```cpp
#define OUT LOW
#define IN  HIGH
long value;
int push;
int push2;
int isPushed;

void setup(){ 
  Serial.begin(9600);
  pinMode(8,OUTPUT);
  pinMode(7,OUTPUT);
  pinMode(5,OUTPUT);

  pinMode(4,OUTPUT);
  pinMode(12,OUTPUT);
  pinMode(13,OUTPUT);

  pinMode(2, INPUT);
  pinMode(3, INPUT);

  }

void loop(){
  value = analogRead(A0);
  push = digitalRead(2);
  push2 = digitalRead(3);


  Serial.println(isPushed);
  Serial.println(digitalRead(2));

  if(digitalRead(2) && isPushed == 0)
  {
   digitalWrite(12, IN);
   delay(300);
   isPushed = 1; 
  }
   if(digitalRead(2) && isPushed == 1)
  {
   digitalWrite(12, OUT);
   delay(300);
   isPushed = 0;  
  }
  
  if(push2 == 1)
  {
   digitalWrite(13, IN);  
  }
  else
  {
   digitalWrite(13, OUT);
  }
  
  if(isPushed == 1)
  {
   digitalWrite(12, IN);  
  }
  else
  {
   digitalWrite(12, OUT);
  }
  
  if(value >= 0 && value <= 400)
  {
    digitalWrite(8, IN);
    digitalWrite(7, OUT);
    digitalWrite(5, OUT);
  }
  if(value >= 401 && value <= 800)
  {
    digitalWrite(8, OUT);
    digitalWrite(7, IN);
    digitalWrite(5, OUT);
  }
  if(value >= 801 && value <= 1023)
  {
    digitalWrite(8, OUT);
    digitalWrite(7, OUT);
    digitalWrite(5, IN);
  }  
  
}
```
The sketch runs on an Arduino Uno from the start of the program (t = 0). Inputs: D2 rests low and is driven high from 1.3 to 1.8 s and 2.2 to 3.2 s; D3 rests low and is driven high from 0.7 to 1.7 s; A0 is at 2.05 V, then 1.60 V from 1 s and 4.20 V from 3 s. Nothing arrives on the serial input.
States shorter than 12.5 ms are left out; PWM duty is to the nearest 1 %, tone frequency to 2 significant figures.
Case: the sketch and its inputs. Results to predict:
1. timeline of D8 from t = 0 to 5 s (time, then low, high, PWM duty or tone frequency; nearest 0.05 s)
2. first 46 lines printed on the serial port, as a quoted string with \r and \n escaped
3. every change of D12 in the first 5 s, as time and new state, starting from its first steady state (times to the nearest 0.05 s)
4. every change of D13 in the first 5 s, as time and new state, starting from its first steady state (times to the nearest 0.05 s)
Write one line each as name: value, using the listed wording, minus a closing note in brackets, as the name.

timeline of D8 from t = 0 to 5 s: 0 s low; 1 s high; 3.4 s low
first 46 lines printed on the serial port, as a quoted string with \r and \n escaped: "0\r\n0\r\n0\r\n0\r\n0\r\n0\r\n0\r\n0\r\n0\r\n0\r\n0\r\n0\r\n0\r\n0\r\n0\r\n0\r\n0\r\n0\r\n0\r\n0\r\n0\r\n0\r\n0\r\n0\r\n0\r\n0\r\n0\r\n0\r\n0\r\n0\r\n0\r\n0\r\n0\r\n0\r\n0\r\n0\r\n0\r\n0\r\n0\r\n0\r\n0\r\n0\r\n0\r\n0\r\n0\r\n0\r\n"
every change of D12 in the first 5 s, as time and new state, starting from its first steady state: 0 s low; 1.3 s high; 1.6 s low; 2.2 s high; 2.5 s low; 2.8 s high; 3.1 s low
every change of D13 in the first 5 s, as time and new state, starting from its first steady state: 0 s low; 0.7 s high; 1.9 s low
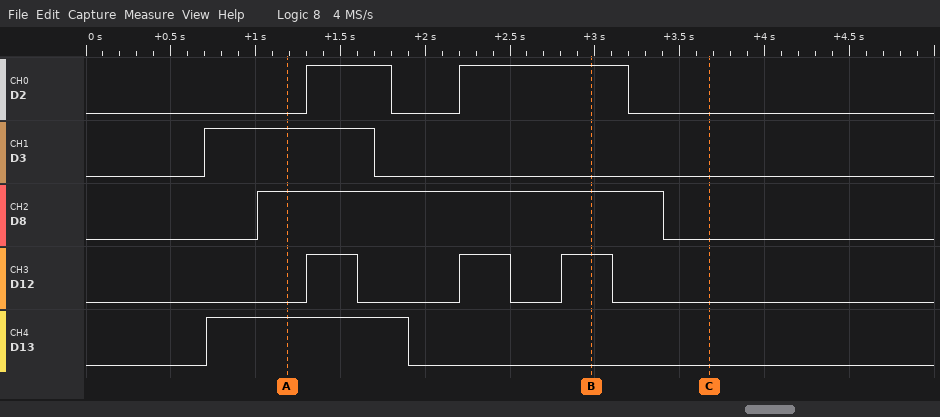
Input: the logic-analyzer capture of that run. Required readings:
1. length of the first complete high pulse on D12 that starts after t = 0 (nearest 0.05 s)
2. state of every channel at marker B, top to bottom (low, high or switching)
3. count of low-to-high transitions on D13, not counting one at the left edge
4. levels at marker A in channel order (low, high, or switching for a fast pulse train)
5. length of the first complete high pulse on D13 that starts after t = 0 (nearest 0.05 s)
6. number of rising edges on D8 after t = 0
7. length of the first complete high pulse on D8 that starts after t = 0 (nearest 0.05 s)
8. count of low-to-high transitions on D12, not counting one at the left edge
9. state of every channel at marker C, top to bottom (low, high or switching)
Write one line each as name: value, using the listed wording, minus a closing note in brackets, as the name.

length of the first complete high pulse on D12 that starts after t = 0: 0.30 s
state of every channel at marker B, top to bottom: D2 high, D3 low, D8 high, D12 high, D13 low
count of low-to-high transitions on D13, not counting one at the left edge: 1
levels at marker A in channel order: D2 low, D3 high, D8 high, D12 low, D13 high
length of the first complete high pulse on D13 that starts after t = 0: 1.20 s
number of rising edges on D8 after t = 0: 1
length of the first complete high pulse on D8 that starts after t = 0: 2.40 s
count of low-to-high transitions on D12, not counting one at the left edge: 3
state of every channel at marker C, top to bottom: D2 low, D3 low, D8 low, D12 low, D13 low
